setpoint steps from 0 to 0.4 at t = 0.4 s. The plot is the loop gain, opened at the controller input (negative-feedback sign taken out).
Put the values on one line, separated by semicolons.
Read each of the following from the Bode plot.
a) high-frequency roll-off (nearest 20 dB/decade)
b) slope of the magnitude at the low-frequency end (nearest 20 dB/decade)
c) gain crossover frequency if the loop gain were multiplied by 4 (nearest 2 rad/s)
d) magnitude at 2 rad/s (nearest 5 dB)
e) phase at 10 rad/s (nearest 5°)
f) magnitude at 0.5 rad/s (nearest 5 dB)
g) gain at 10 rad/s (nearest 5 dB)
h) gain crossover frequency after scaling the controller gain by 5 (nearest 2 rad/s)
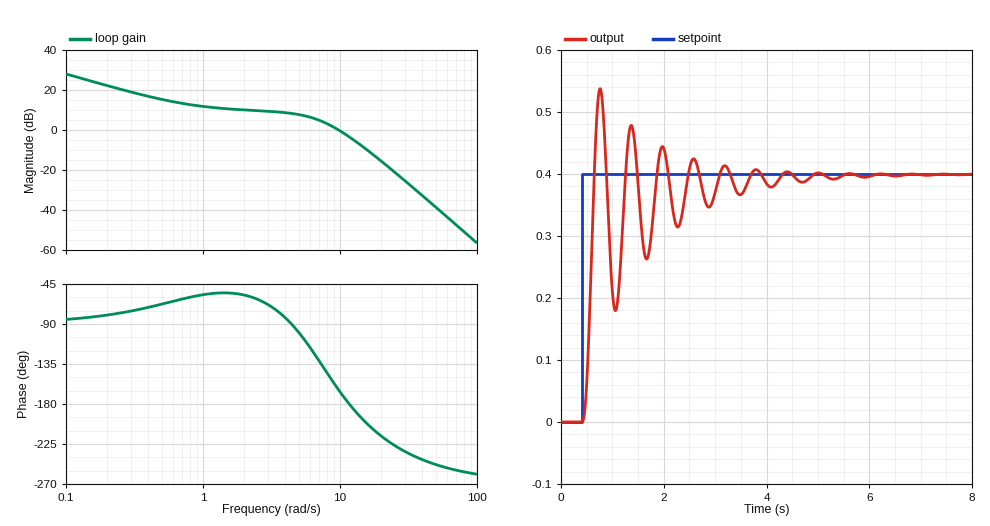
-60 dB/decade; -20 dB/decade; 18 rad/s; 10 dB; -165°; 15 dB; 0 dB; 18 rad/s
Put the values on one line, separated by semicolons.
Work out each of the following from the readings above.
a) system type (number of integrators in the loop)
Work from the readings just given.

1
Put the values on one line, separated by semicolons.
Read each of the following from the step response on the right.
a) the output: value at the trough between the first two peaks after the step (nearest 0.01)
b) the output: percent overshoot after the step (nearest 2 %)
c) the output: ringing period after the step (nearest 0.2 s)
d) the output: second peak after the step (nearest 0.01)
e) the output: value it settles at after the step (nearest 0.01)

0.18; 34 %; 0.6 s; 0.48; 0.40
